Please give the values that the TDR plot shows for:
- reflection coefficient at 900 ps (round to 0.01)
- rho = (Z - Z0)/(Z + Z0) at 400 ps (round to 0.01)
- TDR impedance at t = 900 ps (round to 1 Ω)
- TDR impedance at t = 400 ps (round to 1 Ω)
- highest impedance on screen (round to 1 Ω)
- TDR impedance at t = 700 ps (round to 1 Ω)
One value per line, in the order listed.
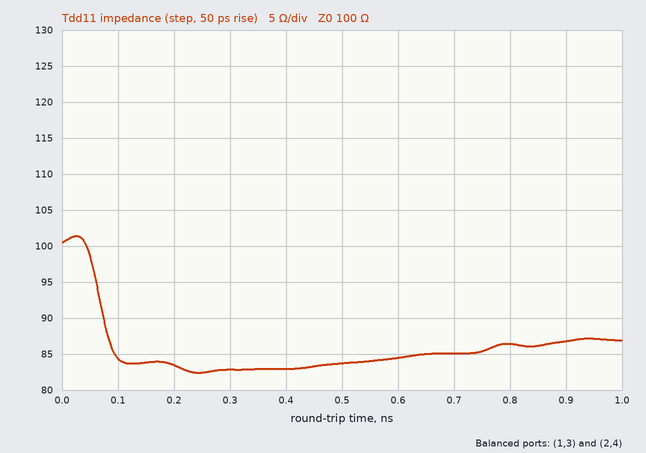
-0.07
-0.09
87 Ω
83 Ω
101 Ω
85 Ω
